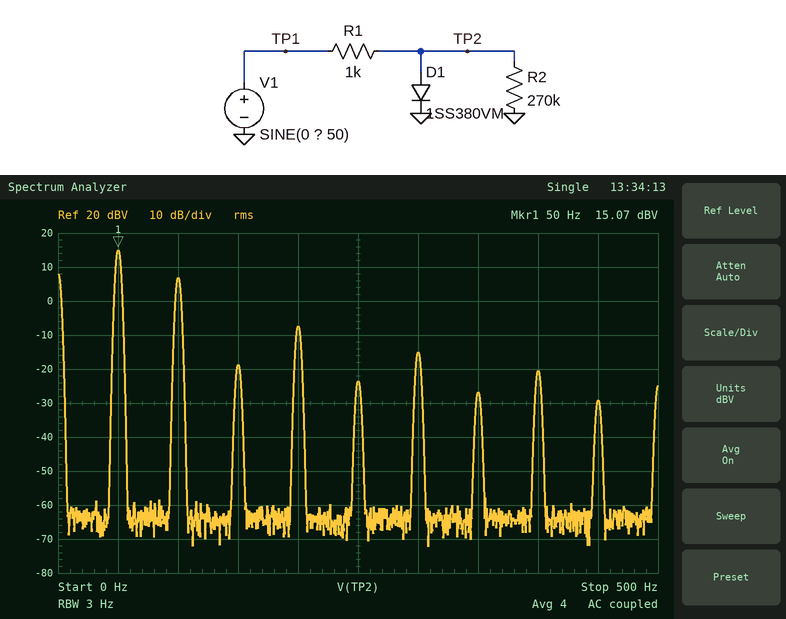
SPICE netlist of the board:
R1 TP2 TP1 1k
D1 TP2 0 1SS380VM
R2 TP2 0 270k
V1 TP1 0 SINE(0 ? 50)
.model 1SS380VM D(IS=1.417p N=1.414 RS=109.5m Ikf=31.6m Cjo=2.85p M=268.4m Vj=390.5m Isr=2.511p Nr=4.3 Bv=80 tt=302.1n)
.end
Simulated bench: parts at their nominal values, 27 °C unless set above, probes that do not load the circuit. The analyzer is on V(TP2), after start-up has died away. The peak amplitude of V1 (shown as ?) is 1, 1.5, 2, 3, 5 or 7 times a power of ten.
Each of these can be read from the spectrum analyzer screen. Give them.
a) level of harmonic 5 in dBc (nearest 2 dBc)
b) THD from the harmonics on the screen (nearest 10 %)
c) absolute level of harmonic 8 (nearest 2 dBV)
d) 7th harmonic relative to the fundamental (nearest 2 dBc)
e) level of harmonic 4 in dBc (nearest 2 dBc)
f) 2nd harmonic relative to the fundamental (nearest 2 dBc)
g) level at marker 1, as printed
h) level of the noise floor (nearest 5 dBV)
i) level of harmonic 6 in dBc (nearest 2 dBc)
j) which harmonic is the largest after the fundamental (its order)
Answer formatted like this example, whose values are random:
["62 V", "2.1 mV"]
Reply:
["-38 dBc", "40 %", "-20 dBV", "-42 dBc", "-22 dBc", "-8 dBc", "15.07 dBV", "-65 dBV", "-30 dBc", "2"]
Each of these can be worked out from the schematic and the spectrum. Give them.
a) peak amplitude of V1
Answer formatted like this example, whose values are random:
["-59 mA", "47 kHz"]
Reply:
["15 V"]
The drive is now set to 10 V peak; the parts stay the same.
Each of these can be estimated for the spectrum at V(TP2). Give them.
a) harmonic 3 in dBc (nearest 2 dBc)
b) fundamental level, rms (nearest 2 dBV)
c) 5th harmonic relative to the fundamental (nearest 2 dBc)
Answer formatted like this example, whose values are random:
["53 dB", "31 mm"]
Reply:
["-30 dBc", "12 dBV", "-36 dBc"]
